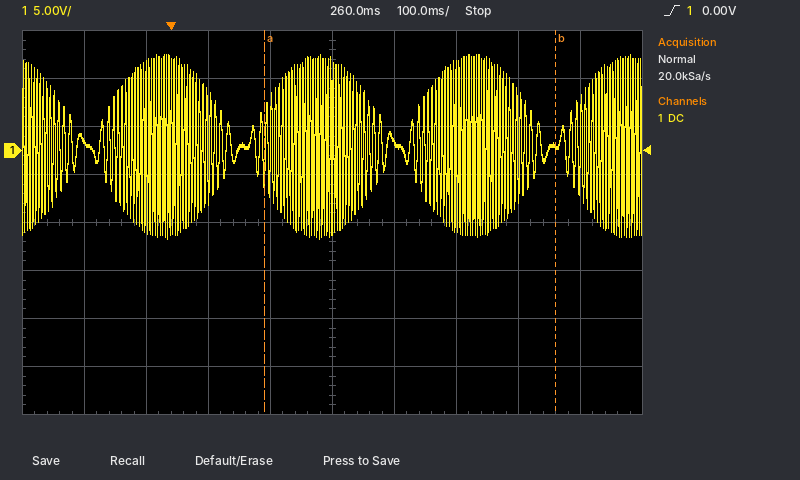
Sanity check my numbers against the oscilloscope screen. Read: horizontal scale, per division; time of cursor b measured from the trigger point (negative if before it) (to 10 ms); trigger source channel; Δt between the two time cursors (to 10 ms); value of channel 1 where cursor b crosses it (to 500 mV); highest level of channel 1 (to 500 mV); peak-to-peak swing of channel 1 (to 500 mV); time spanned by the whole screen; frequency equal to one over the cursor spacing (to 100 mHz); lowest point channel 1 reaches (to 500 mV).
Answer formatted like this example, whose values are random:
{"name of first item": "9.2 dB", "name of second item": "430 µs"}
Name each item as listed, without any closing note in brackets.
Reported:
{"horizontal scale, per division": "100 ms", "time of cursor b measured from the trigger point (negative if before it)": "+620 ms", "trigger source channel": "channel 1", "Δt between the two time cursors": "470 ms", "value of channel 1 where cursor b crosses it": "500 mV", "highest level of channel 1": "10.0 V", "peak-to-peak swing of channel 1": "19.0 V", "time spanned by the whole screen": "1 s", "frequency equal to one over the cursor spacing": "2.1 Hz", "lowest point channel 1 reaches": "-9.0 V"}
